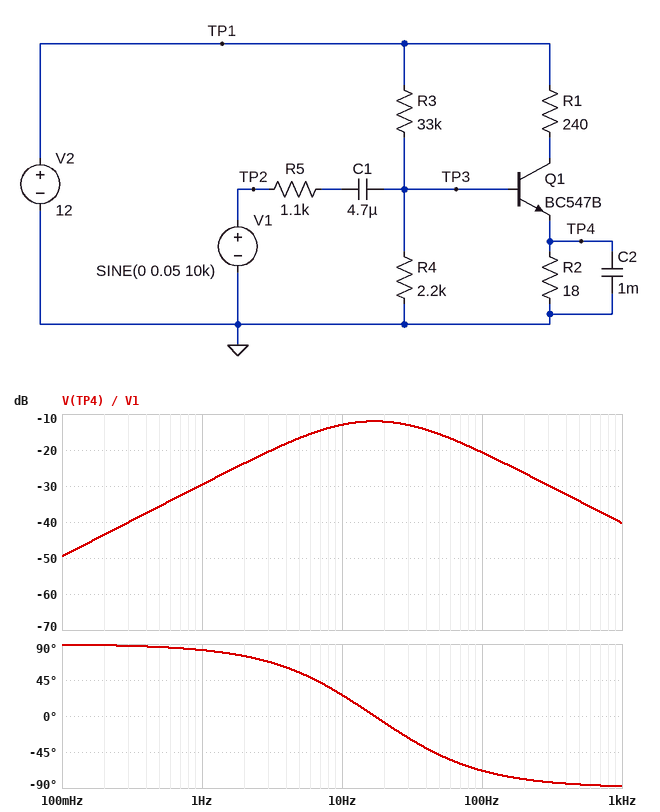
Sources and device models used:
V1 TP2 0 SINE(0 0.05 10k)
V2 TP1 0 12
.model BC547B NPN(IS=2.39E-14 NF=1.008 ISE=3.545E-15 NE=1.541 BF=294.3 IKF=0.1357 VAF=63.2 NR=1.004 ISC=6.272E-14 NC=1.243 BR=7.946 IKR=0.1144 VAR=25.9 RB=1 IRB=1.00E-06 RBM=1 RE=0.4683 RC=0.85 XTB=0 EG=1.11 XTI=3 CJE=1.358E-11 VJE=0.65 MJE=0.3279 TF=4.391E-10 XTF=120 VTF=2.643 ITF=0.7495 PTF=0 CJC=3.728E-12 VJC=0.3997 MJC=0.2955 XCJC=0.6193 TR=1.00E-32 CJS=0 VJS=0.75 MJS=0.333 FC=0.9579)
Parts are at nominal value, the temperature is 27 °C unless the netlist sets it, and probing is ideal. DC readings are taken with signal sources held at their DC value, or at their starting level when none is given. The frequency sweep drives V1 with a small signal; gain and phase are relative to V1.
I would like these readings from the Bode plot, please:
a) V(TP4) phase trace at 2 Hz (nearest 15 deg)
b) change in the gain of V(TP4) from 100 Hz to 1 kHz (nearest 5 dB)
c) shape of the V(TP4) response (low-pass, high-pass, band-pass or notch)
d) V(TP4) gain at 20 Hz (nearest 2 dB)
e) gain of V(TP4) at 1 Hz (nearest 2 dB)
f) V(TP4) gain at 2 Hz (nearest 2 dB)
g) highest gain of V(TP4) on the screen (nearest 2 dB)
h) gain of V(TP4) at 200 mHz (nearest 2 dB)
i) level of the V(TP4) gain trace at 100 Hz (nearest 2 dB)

75 deg
-20 dB
band-pass
-12 dB
-30 dB
-24 dB
-12 dB
-44 dB
-20 dB
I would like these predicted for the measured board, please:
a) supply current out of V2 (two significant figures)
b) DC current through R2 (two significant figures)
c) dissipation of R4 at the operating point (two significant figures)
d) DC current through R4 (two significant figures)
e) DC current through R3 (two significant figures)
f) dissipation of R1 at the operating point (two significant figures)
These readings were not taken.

3.7 mA
3.4 mA
240 µW
330 µA
340 µA
2.7 mW
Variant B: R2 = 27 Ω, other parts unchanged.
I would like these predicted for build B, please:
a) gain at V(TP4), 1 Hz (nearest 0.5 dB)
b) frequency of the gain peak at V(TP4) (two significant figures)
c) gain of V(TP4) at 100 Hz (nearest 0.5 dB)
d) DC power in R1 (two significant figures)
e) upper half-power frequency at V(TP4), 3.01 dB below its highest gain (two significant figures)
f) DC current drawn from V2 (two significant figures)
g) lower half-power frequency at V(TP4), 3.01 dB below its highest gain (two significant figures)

-28.5 dB
15 Hz
-22.0 dB
1.7 mW
38 Hz
3.0 mA
5.7 Hz
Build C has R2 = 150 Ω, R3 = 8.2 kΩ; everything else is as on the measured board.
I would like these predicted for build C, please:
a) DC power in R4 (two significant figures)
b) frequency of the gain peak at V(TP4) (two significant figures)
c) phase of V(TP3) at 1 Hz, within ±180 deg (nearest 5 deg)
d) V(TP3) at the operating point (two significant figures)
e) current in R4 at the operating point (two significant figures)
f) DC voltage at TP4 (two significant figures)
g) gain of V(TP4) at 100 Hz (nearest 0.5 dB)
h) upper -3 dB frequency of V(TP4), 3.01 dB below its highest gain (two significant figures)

2.8 mW
19 Hz
85 deg
2.5 V
1.1 mA
1.8 V
-16.0 dB
57 Hz
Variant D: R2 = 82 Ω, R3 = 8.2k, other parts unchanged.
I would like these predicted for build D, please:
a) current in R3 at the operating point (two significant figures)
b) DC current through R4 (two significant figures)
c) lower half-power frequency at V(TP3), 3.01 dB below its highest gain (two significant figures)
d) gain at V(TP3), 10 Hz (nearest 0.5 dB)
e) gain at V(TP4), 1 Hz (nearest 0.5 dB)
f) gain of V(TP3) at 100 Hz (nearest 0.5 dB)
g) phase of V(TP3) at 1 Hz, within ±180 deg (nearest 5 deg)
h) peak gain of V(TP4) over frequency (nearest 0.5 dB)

1.2 mA
1.1 mA
7.0 Hz
-10.5 dB
-27.0 dB
-11.0 dB
85 deg
-9.5 dB
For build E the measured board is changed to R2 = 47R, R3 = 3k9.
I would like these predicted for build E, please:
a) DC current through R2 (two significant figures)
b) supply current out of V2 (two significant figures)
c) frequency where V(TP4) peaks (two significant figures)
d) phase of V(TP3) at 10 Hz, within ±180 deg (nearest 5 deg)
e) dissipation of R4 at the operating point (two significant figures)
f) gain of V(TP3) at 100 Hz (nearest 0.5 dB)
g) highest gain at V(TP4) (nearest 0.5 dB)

42 mA
44 mA
11 Hz
20 deg
3.5 mW
-45.0 dB
-47.0 dB
